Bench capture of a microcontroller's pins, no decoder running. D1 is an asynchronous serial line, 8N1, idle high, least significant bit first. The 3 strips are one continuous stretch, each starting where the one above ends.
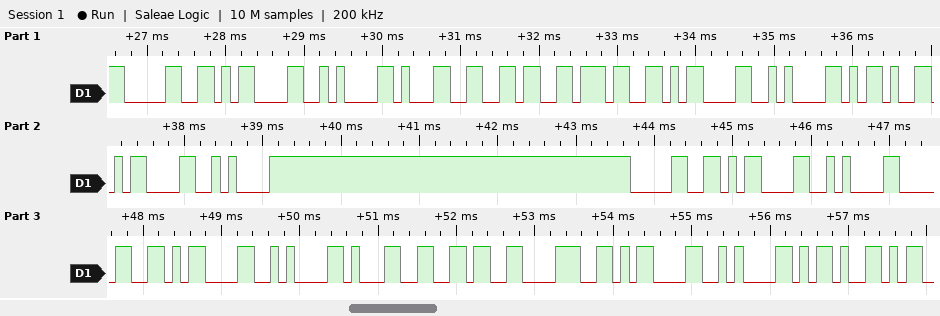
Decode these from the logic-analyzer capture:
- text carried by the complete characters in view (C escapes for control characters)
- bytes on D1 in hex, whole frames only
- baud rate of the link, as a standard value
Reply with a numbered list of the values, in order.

1. "0\r\n167\r\n-\r\n0\r\n0\r\n168\r\n-"
2. 30 0D 0A 31 36 37 0D 0A 2D 0D 0A 30 0D 0A 30 0D 0A 31 36 38 0D 0A 2D
3. 9600 baud
